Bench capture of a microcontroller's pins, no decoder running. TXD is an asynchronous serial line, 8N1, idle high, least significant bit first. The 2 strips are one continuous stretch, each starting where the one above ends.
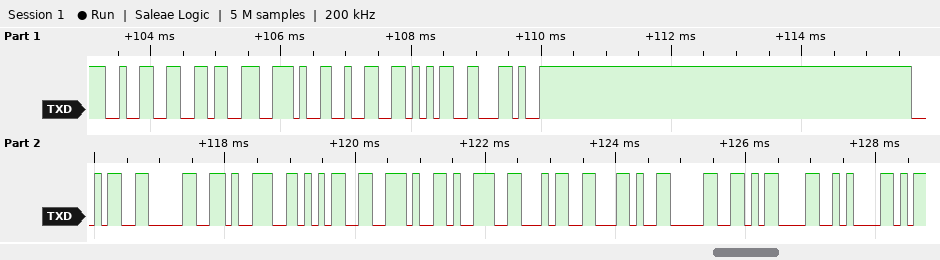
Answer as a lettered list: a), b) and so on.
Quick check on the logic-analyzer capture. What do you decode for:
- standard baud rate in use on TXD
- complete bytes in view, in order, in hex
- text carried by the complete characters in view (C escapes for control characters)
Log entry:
a) 9600 baud
b) 32 36 2E 32 35 2C 34 30 39 35 2E 39 34 2C 30 0D 0A
c) "26.25,4095.94,0\r\n"
